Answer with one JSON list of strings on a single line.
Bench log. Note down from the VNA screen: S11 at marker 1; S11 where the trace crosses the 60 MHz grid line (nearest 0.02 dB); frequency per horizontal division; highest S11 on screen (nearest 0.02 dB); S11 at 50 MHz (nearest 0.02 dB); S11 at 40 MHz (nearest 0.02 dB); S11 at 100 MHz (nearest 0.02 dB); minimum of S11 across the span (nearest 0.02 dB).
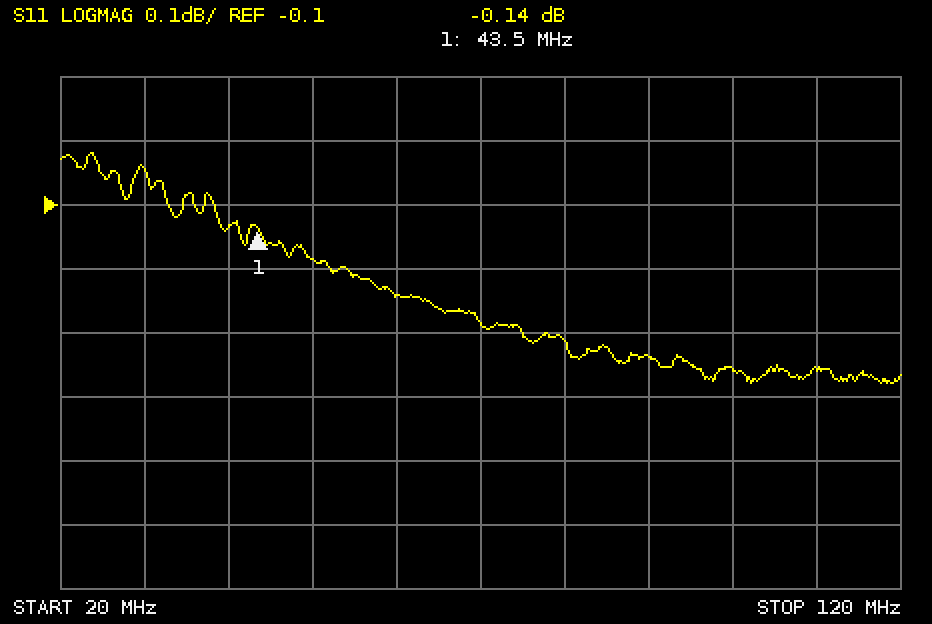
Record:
["-0.14 dB", "-0.24 dB", "10 MHz", "-0.02 dB", "-0.18 dB", "-0.14 dB", "-0.36 dB", "-0.38 dB"]
